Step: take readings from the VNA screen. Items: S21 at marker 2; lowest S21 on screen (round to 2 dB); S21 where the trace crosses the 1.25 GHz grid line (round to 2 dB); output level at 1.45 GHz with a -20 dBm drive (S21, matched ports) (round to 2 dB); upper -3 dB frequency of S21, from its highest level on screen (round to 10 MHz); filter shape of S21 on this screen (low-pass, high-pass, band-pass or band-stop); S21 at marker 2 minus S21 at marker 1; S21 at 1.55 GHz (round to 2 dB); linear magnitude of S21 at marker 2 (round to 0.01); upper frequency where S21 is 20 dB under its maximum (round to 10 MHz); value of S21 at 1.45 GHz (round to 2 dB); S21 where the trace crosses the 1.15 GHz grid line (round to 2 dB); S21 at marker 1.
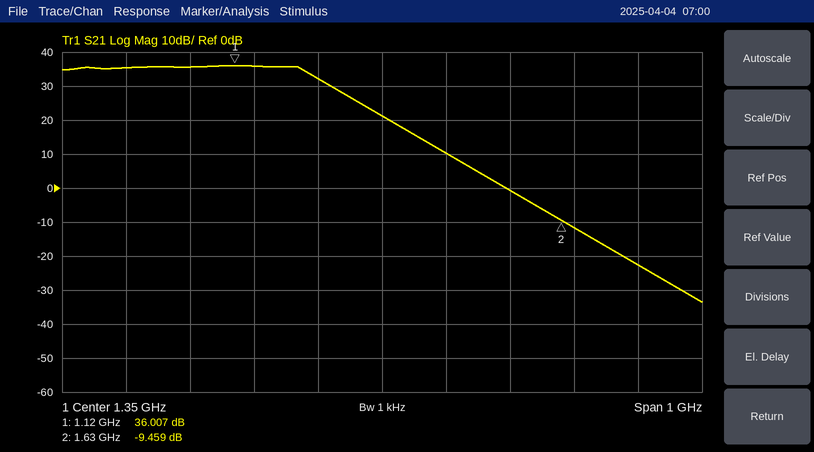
-9.459 dB
-34 dB
32 dB
-10 dBm
1.24 GHz
low-pass
-45.466 dB
0 dB
0.34
1.40 GHz
10 dB
36 dB
36.007 dB
